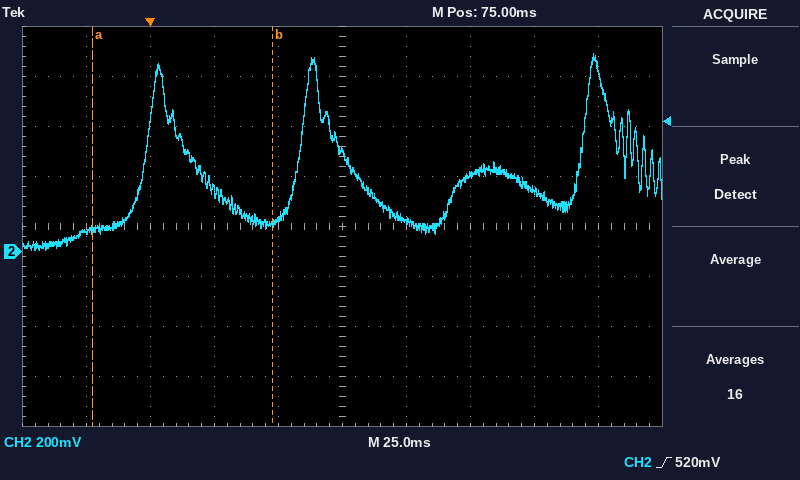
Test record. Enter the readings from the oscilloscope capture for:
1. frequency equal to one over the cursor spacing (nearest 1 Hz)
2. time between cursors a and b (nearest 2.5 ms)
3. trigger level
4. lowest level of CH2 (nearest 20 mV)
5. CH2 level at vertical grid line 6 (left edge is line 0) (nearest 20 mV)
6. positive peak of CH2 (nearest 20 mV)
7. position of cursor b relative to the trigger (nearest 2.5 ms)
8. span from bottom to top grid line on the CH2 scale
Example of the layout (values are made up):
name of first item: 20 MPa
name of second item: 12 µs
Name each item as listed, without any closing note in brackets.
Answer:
frequency equal to one over the cursor spacing: 14 Hz
time between cursors a and b: 70.0 ms
trigger level: 520 mV
lowest level of CH2: 0 mV
CH2 level at vertical grid line 6 (left edge is line 0): 120 mV
positive peak of CH2: 800 mV
position of cursor b relative to the trigger: +47.5 ms
span from bottom to top grid line on the CH2 scale: 1.6 V
